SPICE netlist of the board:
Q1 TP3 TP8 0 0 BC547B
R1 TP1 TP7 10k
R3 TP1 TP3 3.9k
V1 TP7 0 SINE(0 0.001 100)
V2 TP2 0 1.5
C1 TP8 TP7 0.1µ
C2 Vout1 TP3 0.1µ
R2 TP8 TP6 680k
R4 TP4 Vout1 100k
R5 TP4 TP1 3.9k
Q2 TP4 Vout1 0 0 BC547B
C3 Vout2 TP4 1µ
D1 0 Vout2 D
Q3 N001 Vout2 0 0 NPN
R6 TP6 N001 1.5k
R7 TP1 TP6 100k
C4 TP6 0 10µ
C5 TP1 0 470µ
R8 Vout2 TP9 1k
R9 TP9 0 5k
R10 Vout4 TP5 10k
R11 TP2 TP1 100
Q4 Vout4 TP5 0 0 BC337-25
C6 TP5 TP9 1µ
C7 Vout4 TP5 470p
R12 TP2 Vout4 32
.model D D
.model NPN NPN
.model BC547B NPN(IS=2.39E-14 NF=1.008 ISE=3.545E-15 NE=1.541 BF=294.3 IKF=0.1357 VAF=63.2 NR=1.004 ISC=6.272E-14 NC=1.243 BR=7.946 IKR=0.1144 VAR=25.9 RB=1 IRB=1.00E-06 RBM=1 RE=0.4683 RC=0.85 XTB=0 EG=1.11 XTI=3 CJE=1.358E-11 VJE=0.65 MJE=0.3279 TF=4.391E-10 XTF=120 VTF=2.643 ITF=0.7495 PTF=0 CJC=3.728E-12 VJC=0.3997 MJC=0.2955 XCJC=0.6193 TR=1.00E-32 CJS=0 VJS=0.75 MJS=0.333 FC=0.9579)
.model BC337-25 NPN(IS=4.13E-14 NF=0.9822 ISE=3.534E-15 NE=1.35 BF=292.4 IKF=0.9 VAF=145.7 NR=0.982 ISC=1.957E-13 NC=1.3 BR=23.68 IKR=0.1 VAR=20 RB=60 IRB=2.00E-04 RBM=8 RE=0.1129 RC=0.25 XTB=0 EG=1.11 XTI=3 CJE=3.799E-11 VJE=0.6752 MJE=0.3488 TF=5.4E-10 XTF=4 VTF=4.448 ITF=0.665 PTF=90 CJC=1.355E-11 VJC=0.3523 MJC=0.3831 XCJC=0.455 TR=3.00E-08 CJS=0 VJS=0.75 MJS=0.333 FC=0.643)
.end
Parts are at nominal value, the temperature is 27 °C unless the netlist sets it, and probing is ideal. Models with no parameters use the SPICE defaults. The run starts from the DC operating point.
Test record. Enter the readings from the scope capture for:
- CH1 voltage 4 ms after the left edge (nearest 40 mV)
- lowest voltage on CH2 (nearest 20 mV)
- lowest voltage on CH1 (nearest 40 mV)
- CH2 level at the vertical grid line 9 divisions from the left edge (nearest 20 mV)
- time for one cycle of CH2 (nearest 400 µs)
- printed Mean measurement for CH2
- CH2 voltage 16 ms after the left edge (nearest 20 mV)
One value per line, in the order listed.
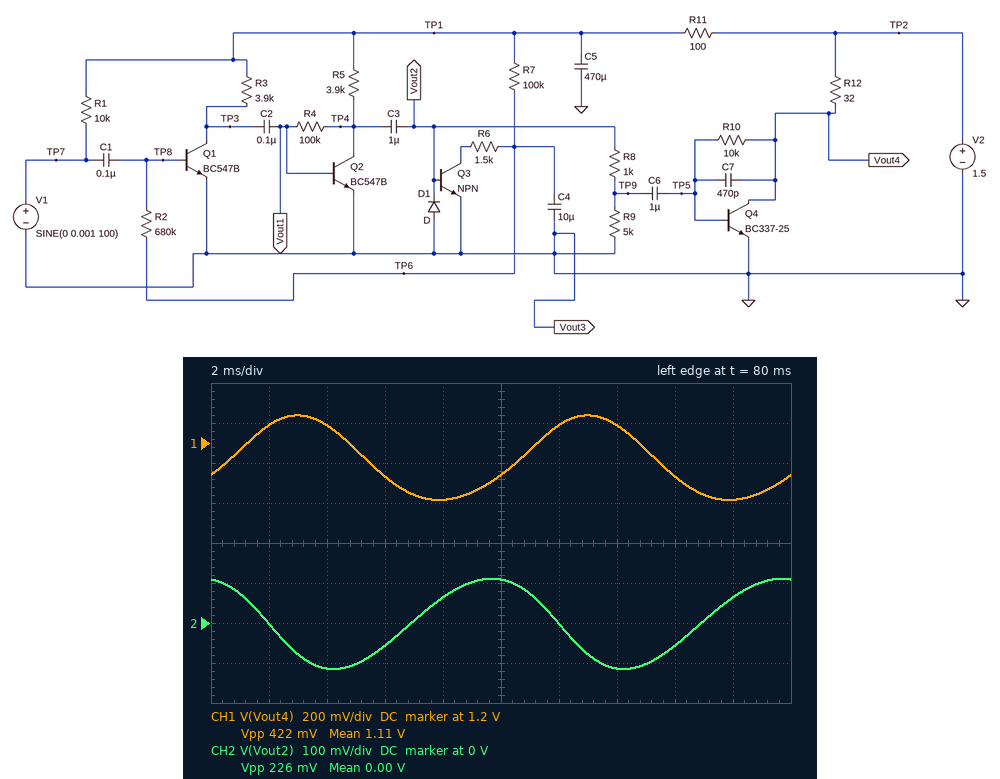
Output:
1.28 V
-120 mV
920 mV
60 mV
10.0 ms
0.00 V
-60 mV
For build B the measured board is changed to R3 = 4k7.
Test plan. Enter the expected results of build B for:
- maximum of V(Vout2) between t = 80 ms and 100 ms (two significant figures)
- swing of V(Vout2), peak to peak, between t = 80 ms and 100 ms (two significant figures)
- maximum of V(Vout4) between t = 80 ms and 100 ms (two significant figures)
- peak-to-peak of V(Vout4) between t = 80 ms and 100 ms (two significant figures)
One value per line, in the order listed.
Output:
55 mV
98 mV
1.2 V
190 mV
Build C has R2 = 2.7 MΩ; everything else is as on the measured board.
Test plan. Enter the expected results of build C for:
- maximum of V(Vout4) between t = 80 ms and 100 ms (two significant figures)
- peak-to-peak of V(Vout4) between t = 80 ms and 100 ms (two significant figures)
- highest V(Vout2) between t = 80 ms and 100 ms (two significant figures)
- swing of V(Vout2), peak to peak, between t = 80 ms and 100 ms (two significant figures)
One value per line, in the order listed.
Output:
1.2 V
160 mV
42 mV
84 mV
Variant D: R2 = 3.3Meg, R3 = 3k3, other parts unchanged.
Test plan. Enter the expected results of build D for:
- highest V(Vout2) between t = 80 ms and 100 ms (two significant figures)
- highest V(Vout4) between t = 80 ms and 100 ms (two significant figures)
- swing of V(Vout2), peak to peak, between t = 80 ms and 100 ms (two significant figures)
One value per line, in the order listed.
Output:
30 mV
1.2 V
61 mV
